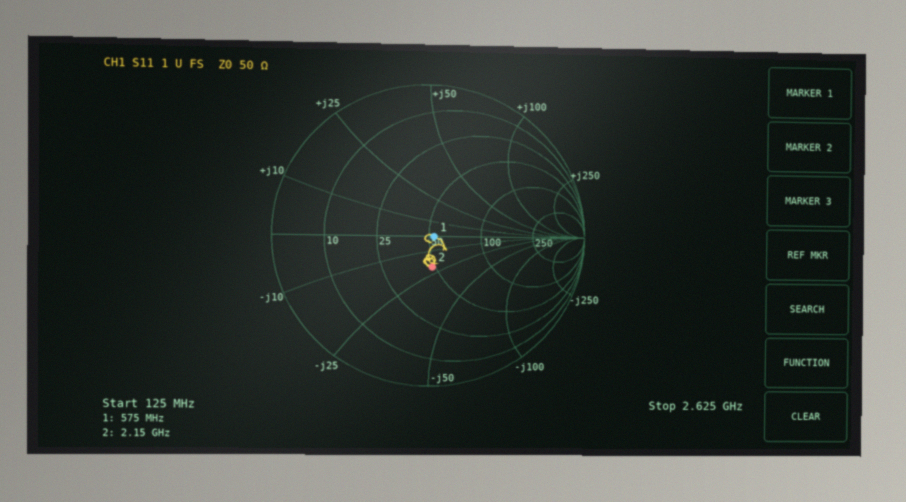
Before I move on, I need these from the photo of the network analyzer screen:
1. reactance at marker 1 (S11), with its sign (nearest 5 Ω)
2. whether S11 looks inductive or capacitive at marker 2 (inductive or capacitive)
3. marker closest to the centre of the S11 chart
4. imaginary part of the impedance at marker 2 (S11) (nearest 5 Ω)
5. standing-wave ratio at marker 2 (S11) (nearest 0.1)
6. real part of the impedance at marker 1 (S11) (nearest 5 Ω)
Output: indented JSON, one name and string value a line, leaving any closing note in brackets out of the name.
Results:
{
  "reactance at marker 1 (S11), with its sign": "0 Ω",
  "whether S11 looks inductive or capacitive at marker 2": "capacitive",
  "marker closest to the centre of the S11 chart": "marker 1",
  "imaginary part of the impedance at marker 2 (S11)": "-20 Ω",
  "standing-wave ratio at marker 2 (S11)": "1.5",
  "real part of the impedance at marker 1 (S11)": "55 Ω"
}
